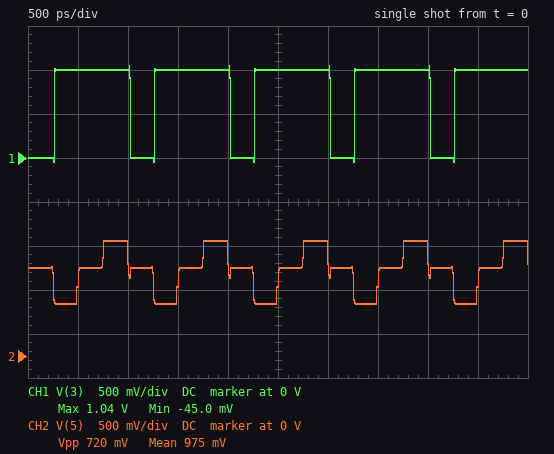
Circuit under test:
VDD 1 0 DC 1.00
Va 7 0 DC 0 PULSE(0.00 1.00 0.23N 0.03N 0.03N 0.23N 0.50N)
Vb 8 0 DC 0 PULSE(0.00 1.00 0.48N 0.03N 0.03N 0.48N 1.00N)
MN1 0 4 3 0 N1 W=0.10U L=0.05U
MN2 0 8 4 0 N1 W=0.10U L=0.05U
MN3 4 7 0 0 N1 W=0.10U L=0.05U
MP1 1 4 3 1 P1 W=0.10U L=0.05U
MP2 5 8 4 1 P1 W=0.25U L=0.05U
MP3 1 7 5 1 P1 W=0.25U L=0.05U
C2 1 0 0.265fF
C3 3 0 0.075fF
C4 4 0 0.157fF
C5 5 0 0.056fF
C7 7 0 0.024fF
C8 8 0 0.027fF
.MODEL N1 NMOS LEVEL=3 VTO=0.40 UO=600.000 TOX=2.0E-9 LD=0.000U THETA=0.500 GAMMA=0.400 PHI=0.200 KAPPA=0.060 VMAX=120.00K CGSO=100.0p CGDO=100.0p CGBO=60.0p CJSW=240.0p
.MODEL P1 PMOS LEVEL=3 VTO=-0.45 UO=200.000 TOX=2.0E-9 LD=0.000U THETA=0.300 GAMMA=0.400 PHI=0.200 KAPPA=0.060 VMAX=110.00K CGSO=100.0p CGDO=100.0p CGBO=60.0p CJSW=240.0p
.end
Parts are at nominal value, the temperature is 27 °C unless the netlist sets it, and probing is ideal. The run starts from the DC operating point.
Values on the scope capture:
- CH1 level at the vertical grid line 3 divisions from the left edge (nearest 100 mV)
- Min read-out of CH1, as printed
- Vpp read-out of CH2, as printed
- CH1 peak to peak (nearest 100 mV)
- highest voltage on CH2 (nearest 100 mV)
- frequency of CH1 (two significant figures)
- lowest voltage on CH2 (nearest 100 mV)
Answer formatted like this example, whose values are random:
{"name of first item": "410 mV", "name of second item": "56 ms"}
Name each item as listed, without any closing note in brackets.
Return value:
{"CH1 level at the vertical grid line 3 divisions from the left edge": "1.0 V", "Min read-out of CH1, as printed": "-45.0 mV", "Vpp read-out of CH2, as printed": "720 mV", "CH1 peak to peak": "1.1 V", "highest voltage on CH2": "1.3 V", "frequency of CH1": "1.0 GHz", "lowest voltage on CH2": "600 mV"}
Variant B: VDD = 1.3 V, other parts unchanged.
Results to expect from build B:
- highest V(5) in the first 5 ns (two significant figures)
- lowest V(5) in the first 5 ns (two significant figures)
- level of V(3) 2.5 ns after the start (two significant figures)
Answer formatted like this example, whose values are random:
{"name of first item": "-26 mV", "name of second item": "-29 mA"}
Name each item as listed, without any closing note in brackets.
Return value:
{"highest V(5) in the first 5 ns": "1.4 V", "lowest V(5) in the first 5 ns": "640 mV", "level of V(3) 2.5 ns after the start": "1.3 V"}
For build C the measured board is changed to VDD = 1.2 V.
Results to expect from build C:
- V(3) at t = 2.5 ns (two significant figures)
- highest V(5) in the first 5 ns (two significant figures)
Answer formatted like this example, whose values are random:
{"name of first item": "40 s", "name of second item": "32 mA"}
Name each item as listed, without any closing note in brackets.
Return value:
{"V(3) at t = 2.5 ns": "1.2 V", "highest V(5) in the first 5 ns": "1.4 V"}
